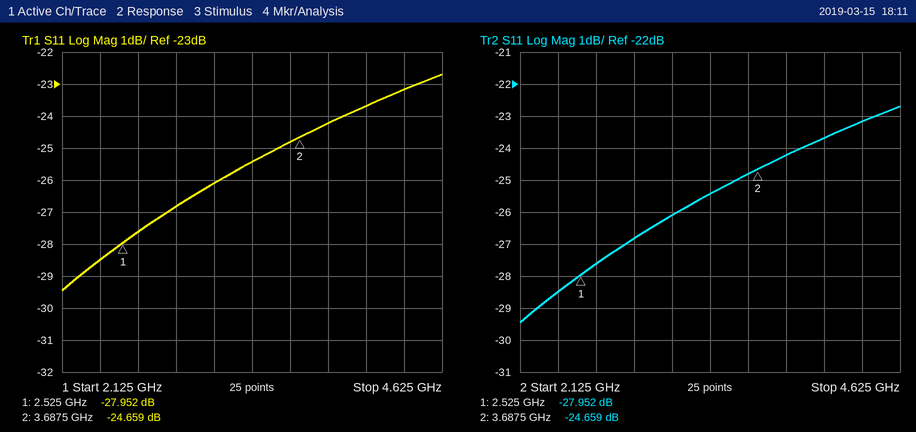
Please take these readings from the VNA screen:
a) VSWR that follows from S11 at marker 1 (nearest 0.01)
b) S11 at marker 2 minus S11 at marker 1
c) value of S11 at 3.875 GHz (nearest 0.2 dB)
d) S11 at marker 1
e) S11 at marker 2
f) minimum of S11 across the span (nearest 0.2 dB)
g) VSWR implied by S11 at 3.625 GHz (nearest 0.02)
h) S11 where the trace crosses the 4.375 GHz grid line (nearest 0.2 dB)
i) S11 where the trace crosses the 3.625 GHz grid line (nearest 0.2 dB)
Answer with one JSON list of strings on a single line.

["1.08", "3.293 dB", "-24.2 dB", "-27.952 dB", "-24.659 dB", "-29.4 dB", "1.12", "-23.2 dB", "-24.8 dB"]
